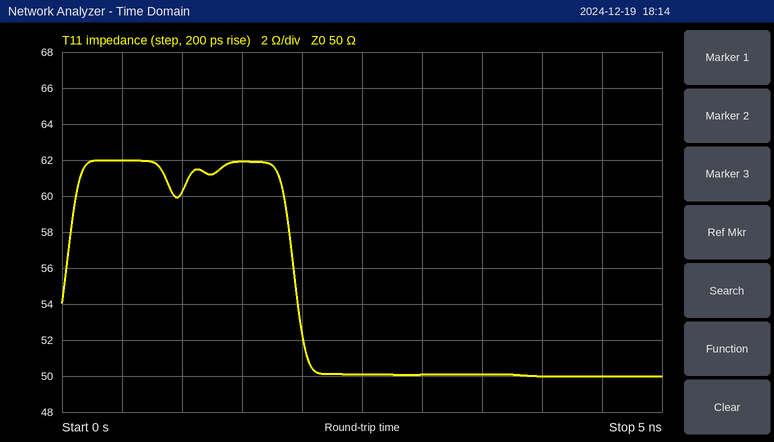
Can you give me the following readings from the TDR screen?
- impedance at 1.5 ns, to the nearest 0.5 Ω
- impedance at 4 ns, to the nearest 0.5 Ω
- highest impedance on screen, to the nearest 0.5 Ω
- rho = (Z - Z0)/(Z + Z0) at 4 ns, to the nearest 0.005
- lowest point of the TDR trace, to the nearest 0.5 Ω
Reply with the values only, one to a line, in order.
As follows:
62.0 Ω
50.0 Ω
62.0 Ω
0.000
50.0 Ω
